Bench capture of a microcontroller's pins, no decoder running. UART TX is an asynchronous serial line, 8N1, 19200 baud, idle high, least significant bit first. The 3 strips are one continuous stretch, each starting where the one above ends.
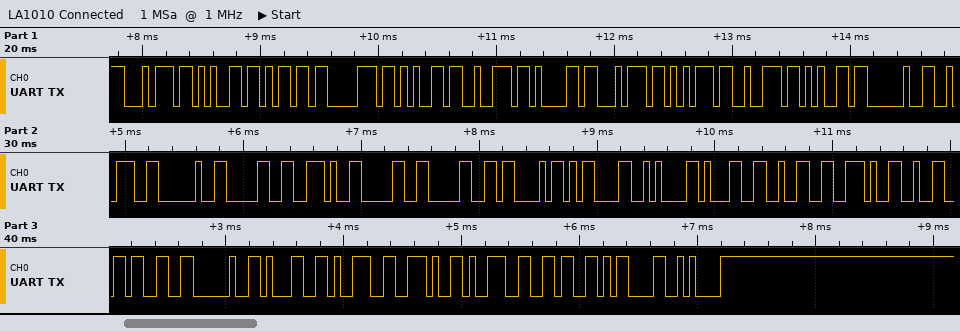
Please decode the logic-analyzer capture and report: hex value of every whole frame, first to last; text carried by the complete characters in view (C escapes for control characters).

0x74 0x65 0x6D 0x70 0x65 0x72 0x61 0x74 0x75 0x72 0x65 0x20 0x3A 0x20 0x30 0x2E 0x30 0x30 0x43 0x0D 0x0A 0x31 0x32 0x2E 0x32 0x33 0x20 0x31 0x39 0x2E 0x39 0x36 0x0D 0x0A
"temperature : 0.00C\r\n12.23 19.96\r\n"
